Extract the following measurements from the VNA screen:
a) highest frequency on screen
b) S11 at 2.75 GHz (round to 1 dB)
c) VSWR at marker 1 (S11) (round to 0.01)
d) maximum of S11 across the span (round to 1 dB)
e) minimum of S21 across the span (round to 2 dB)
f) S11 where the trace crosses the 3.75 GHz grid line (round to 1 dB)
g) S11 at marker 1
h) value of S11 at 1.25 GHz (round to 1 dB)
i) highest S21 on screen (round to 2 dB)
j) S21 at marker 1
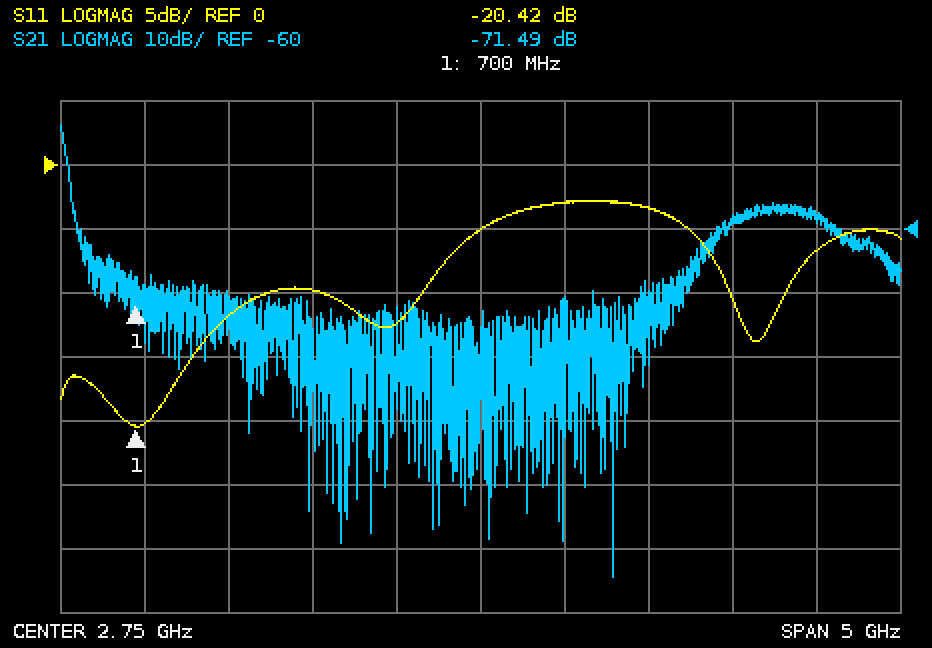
5.25 GHz
-5 dB
1.21
-3 dB
-114 dB
-3 dB
-20.42 dB
-12 dB
-44 dB
-71.49 dB
